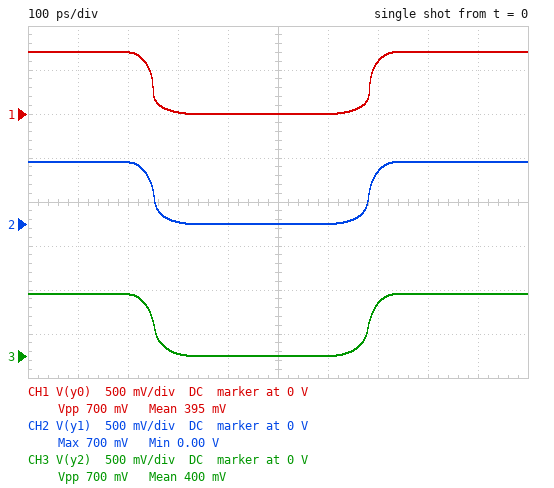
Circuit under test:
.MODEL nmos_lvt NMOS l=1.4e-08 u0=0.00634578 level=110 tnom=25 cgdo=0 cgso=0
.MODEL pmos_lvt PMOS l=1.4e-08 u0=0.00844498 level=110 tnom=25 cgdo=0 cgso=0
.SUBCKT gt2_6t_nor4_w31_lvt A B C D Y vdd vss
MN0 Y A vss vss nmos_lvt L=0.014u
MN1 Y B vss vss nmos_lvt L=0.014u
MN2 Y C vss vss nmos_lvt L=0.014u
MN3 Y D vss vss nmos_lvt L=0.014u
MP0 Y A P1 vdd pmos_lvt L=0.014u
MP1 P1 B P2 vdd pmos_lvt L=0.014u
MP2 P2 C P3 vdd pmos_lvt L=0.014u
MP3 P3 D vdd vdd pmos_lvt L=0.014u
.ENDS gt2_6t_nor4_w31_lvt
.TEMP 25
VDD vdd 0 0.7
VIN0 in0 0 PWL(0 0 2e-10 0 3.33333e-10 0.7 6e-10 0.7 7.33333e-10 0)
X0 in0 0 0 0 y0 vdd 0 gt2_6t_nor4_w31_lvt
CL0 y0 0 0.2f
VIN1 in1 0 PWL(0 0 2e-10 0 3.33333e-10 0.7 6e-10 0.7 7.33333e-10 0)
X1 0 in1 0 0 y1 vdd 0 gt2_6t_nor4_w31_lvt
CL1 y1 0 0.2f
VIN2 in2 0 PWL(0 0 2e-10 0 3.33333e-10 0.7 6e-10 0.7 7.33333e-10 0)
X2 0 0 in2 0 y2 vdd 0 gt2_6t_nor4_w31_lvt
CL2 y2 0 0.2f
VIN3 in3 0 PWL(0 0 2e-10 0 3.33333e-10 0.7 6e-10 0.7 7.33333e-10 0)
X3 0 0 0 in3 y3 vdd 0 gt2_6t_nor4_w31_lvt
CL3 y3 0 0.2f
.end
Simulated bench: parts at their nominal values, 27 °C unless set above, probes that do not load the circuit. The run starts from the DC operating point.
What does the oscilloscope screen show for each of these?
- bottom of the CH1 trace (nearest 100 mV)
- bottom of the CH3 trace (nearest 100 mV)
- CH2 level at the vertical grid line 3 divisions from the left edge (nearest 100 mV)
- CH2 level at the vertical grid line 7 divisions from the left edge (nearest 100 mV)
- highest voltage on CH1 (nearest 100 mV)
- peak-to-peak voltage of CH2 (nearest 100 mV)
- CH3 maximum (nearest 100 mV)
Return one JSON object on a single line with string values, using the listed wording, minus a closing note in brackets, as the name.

{"bottom of the CH1 trace": "0 V", "bottom of the CH3 trace": "0 V", "CH2 level at the vertical grid line 3 divisions from the left edge": "0 V", "CH2 level at the vertical grid line 7 divisions from the left edge": "600 mV", "highest voltage on CH1": "700 mV", "peak-to-peak voltage of CH2": "700 mV", "CH3 maximum": "700 mV"}
